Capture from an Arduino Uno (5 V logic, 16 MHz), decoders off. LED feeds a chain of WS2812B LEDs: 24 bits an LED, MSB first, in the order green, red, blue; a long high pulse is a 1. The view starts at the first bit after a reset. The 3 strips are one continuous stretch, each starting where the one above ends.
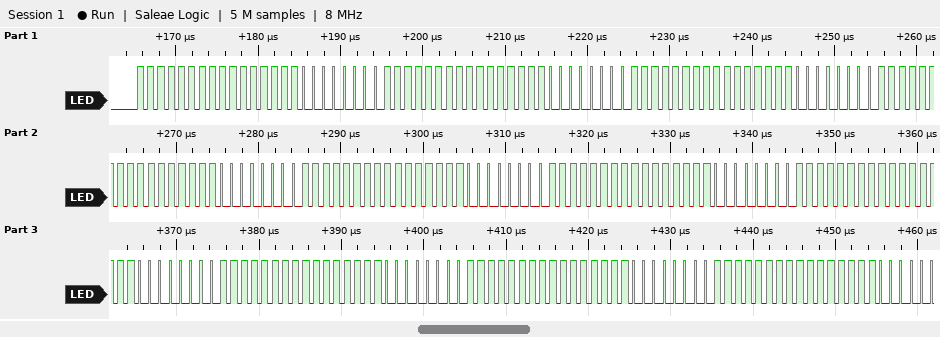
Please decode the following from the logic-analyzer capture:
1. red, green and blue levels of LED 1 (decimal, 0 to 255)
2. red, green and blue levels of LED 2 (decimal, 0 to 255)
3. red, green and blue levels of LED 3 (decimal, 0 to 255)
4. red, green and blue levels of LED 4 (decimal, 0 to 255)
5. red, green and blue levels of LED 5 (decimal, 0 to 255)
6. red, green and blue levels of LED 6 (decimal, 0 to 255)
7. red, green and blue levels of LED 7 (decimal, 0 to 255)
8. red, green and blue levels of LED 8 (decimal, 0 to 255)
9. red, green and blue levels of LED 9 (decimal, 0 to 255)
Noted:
255, 255, 0
255, 255, 0
255, 255, 0
255, 255, 0
255, 255, 0
255, 255, 0
255, 255, 0
255, 255, 0
255, 255, 0
